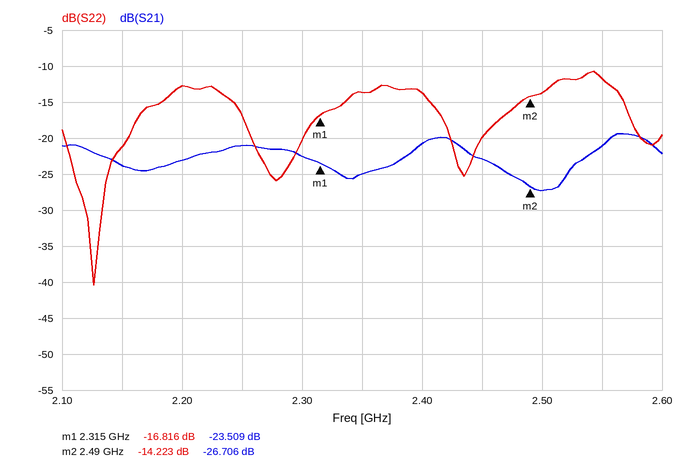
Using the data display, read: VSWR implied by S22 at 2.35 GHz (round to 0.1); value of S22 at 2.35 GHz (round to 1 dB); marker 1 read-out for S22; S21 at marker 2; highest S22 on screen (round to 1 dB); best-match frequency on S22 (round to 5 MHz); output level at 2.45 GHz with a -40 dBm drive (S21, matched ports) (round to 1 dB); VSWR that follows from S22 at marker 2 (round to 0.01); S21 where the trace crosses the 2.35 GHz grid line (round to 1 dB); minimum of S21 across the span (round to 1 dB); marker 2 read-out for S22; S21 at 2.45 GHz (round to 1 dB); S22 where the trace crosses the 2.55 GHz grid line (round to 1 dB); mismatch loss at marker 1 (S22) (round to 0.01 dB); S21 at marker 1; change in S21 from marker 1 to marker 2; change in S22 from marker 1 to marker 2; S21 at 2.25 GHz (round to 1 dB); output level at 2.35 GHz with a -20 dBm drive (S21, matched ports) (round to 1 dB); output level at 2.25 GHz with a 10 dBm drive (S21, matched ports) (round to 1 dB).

1.5
-14 dB
-16.816 dB
-26.706 dB
-11 dB
2.125 GHz
-63 dBm
1.48
-25 dB
-27 dB
-14.223 dB
-23 dB
-12 dB
0.09 dB
-23.509 dB
-3.197 dB
2.593 dB
-21 dB
-45 dBm
-11 dBm
